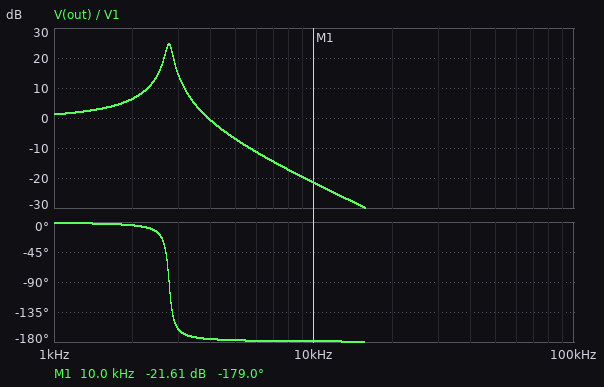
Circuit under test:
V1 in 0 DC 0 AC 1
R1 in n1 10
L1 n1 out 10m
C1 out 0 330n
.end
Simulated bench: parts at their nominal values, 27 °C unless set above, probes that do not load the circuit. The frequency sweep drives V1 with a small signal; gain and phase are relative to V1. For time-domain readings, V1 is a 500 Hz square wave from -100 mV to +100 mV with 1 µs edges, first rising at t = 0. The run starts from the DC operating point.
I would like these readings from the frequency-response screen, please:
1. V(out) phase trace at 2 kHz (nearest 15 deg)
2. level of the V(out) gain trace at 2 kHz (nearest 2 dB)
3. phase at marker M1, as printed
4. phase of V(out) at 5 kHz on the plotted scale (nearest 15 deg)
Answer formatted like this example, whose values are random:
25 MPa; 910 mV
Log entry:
0 deg; 6 dB; -179.0 deg; -180 deg
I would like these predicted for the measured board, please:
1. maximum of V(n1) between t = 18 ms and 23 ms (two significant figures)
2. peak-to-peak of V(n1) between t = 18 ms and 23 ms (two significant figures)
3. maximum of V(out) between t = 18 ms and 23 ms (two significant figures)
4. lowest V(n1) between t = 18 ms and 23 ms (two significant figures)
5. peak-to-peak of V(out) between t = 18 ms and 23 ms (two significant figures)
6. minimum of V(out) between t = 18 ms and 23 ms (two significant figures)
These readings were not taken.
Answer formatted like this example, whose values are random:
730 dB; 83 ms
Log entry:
110 mV; 220 mV; 250 mV; -110 mV; 500 mV; -250 mV
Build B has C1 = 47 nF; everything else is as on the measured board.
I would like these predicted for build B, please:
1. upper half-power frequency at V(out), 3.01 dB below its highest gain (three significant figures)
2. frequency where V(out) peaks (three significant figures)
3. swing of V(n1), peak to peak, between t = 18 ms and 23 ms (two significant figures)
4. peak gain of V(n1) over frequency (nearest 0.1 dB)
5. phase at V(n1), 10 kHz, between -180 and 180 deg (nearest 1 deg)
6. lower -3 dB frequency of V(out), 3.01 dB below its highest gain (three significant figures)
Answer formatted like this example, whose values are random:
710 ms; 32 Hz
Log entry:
7.42 kHz; 7.34 kHz; 210 mV; 0 dB; 2 deg; 7.26 kHz
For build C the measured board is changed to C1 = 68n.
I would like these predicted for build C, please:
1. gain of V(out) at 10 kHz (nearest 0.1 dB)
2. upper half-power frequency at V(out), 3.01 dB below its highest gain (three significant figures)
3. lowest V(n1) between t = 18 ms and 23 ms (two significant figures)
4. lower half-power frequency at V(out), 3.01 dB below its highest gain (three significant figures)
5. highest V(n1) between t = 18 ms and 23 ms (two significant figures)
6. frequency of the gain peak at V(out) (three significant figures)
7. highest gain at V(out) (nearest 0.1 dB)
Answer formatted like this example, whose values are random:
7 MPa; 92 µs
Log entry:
-4.5 dB; 6.18 kHz; -100 mV; 6.02 kHz; 100 mV; 6.10 kHz; 31.7 dB
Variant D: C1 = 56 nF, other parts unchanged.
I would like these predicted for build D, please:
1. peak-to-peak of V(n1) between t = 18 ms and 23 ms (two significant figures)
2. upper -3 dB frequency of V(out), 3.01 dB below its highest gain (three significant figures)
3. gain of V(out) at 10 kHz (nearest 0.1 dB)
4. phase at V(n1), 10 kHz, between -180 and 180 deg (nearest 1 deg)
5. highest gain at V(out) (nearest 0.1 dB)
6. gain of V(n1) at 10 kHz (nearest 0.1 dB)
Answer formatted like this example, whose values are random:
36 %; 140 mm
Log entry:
210 mV; 6.80 kHz; -1.7 dB; 2 deg; 32.5 dB; 0 dB
